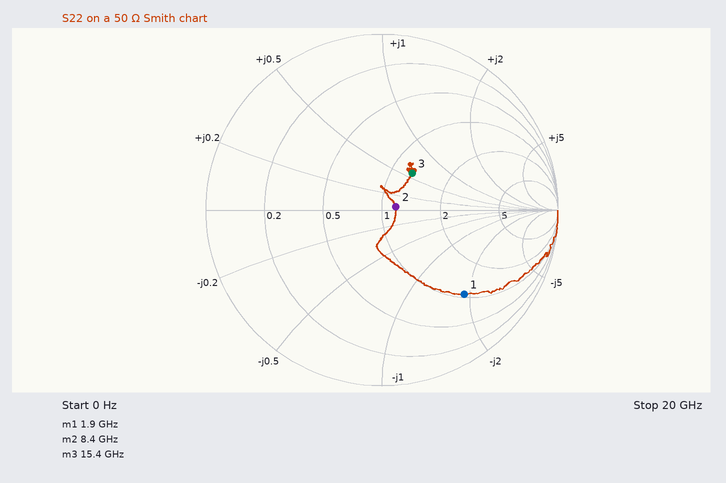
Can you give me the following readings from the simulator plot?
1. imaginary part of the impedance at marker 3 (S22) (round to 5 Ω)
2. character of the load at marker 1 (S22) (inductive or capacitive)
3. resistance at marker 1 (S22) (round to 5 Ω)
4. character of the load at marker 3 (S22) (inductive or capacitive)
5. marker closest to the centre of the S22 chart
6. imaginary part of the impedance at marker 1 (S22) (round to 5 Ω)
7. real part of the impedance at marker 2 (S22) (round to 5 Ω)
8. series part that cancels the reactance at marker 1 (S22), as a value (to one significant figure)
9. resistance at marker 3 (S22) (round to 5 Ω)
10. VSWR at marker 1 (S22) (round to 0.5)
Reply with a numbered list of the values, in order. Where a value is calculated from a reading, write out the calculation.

1. +30 Ω
2. capacitive
3. 55 Ω
4. inductive
5. marker 2
6. -95 Ω
7. 60 Ω
8. L = 95 Ω/(2π × 1.9 GHz) ≈ 8 nH
9. 65 Ω
10. 5.0
